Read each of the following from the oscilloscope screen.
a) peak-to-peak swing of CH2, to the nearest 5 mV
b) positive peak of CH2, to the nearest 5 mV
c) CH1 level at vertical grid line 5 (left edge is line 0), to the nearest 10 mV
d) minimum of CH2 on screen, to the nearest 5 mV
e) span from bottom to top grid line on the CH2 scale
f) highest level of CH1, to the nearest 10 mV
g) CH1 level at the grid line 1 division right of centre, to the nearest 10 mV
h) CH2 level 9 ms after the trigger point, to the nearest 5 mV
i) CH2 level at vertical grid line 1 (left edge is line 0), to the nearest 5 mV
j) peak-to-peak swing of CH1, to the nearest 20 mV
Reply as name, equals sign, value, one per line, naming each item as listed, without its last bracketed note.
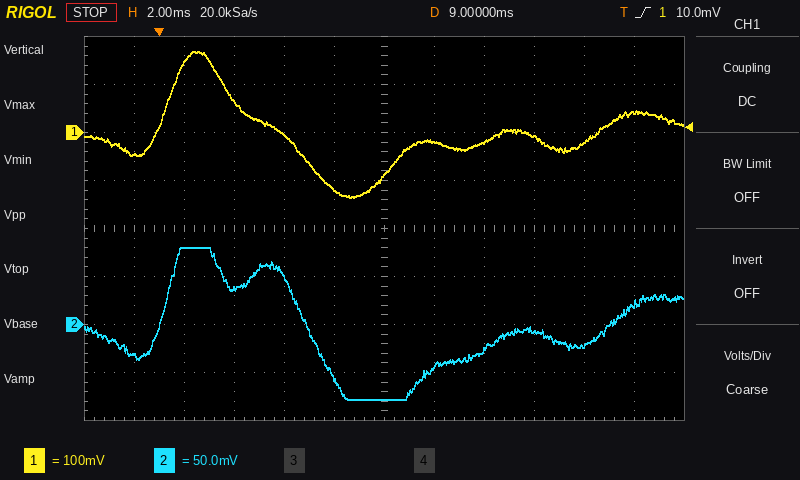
peak-to-peak swing of CH2, to the nearest 5 mV = 160 mV
positive peak of CH2, to the nearest 5 mV = 80 mV
CH1 level at vertical grid line 5 (left edge is line 0), to the nearest 10 mV = -120 mV
minimum of CH2 on screen, to the nearest 5 mV = -80 mV
span from bottom to top grid line on the CH2 scale = 400 mV
highest level of CH1, to the nearest 10 mV = 170 mV
CH1 level at the grid line 1 division right of centre, to the nearest 10 mV = -20 mV
CH2 level 9 ms after the trigger point, to the nearest 5 mV = -80 mV
CH2 level at vertical grid line 1 (left edge is line 0), to the nearest 5 mV = -35 mV
peak-to-peak swing of CH1, to the nearest 20 mV = 300 mV
